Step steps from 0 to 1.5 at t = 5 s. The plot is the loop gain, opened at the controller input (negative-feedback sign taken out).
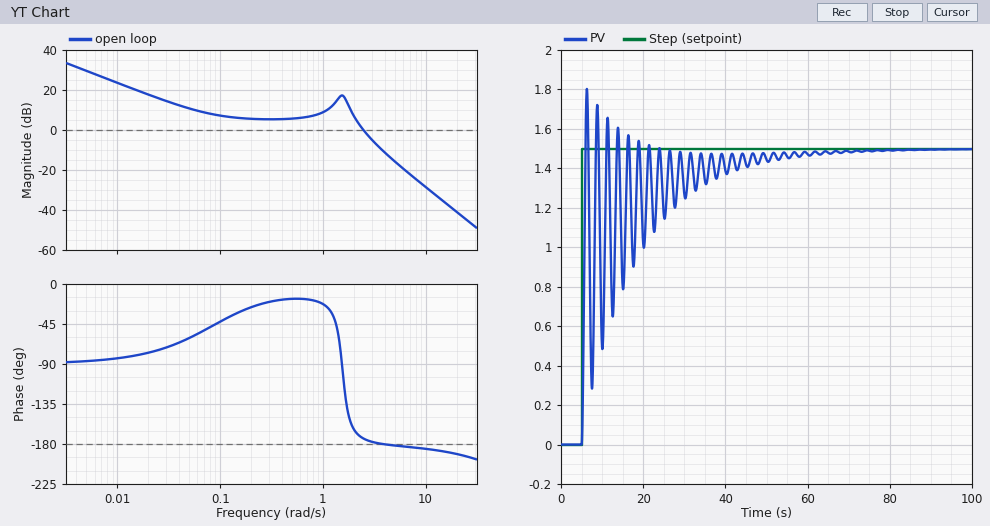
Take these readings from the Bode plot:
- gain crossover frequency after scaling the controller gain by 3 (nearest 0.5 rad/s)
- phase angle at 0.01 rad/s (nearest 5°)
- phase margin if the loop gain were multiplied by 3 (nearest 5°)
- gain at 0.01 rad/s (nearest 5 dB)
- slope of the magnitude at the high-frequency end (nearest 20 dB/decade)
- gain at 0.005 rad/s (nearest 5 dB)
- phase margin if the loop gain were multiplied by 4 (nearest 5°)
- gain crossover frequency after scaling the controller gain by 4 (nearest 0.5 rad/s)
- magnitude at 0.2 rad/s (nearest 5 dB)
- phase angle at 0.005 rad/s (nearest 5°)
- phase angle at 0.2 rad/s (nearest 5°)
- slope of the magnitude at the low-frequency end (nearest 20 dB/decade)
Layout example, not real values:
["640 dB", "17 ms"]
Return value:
["3.5 rad/s", "-85°", "0°", "25 dB", "-40 dB/decade", "30 dB", "0°", "4.0 rad/s", "5 dB", "-85°", "-25°", "-20 dB/decade"]
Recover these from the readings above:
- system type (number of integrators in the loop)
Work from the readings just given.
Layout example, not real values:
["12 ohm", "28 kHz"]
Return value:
["1"]
